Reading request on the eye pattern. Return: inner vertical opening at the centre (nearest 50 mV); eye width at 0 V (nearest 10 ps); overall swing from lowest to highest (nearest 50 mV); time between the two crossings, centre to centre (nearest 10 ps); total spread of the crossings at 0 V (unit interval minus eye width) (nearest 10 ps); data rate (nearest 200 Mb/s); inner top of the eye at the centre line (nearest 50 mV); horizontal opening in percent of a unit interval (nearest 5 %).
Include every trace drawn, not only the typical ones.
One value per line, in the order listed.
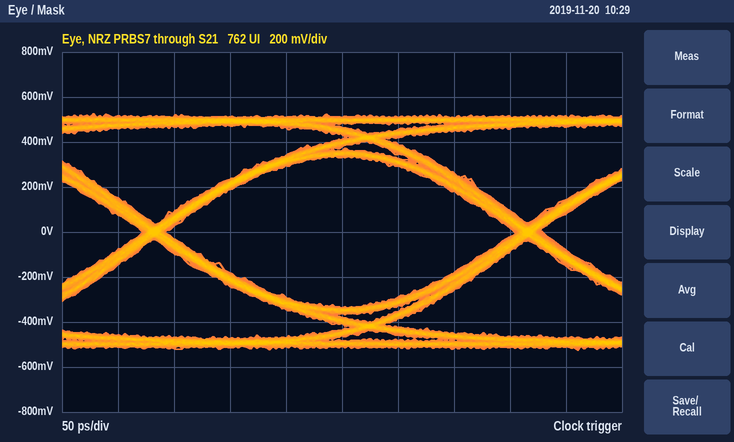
650 mV
310 ps
1.05 V
330 ps
20 ps
3.0 Gb/s
350 mV
95 %
